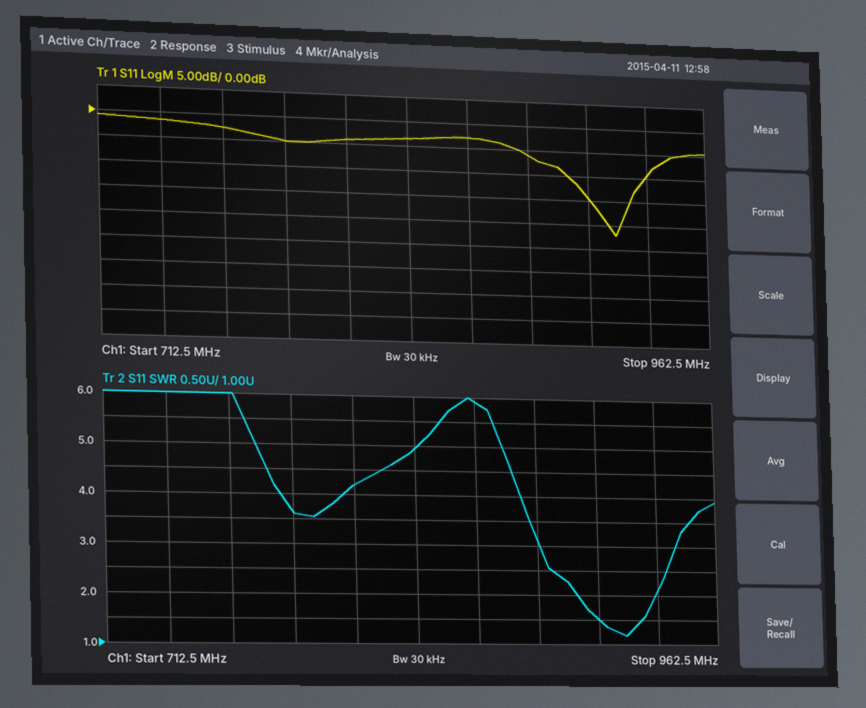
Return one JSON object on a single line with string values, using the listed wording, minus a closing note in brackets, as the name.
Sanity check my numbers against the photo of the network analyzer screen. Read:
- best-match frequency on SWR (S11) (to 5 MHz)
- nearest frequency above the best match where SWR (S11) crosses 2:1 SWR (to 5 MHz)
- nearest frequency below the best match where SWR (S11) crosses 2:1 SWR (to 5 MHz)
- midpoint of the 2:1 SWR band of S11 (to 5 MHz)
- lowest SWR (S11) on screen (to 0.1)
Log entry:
{"best-match frequency on SWR (S11)": "925 MHz", "nearest frequency above the best match where SWR (S11) crosses 2:1 SWR": "935 MHz", "nearest frequency below the best match where SWR (S11) crosses 2:1 SWR": "905 MHz", "midpoint of the 2:1 SWR band of S11": "920 MHz", "lowest SWR (S11) on screen": "1.2"}
